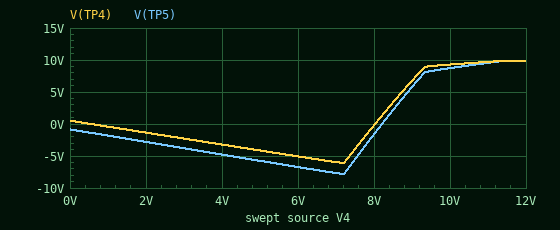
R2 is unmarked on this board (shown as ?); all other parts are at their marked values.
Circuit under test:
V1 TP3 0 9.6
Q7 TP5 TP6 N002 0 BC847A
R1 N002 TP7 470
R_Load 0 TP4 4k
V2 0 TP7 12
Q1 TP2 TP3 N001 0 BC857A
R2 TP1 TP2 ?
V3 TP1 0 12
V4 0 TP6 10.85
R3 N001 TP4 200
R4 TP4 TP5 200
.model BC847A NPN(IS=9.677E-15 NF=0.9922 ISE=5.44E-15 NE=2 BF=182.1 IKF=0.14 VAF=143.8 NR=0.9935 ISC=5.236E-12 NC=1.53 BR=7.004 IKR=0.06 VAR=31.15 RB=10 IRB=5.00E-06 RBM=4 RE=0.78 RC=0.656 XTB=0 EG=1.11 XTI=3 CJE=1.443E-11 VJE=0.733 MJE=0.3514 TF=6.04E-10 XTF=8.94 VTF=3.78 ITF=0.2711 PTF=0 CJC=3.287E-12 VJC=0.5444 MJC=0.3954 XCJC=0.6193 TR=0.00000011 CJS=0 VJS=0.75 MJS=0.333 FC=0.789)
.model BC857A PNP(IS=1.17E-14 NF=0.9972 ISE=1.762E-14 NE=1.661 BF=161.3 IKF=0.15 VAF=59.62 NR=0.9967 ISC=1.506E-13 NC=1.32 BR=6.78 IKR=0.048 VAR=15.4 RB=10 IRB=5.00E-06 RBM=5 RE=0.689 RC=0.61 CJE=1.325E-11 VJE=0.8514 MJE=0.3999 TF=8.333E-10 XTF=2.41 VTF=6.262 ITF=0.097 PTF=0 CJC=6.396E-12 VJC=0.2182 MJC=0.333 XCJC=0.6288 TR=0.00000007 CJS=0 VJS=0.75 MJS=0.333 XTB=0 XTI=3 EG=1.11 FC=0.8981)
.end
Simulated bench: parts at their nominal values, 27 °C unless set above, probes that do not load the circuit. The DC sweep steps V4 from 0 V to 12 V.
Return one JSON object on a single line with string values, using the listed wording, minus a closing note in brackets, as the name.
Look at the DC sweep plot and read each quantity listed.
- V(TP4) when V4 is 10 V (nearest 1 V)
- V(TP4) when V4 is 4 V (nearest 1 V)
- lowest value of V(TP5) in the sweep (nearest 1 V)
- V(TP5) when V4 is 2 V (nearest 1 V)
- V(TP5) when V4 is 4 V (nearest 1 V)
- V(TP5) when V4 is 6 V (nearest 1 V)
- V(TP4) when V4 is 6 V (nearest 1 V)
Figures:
{"V(TP4) when V4 is 10 V": "9 V", "V(TP4) when V4 is 4 V": "-3 V", "lowest value of V(TP5) in the sweep": "-8 V", "V(TP5) when V4 is 2 V": "-3 V", "V(TP5) when V4 is 4 V": "-5 V", "V(TP5) when V4 is 6 V": "-7 V", "V(TP4) when V4 is 6 V": "-5 V"}
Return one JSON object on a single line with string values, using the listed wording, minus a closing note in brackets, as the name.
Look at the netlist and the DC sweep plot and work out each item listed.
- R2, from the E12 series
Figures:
{"R2, from the E12 series": "220 Ω"}
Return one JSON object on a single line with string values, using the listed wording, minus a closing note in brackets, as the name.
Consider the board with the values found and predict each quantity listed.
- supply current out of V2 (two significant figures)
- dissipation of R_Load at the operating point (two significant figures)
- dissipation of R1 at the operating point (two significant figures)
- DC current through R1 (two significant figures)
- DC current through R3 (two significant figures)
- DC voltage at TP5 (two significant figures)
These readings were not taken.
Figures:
{"supply current out of V2": "1.1 mA", "dissipation of R_Load at the operating point": "23 mW", "dissipation of R1 at the operating point": "530 µW", "DC current through R1": "1.1 mA", "DC current through R3": "3.5 mA", "DC voltage at TP5": "9.4 V"}
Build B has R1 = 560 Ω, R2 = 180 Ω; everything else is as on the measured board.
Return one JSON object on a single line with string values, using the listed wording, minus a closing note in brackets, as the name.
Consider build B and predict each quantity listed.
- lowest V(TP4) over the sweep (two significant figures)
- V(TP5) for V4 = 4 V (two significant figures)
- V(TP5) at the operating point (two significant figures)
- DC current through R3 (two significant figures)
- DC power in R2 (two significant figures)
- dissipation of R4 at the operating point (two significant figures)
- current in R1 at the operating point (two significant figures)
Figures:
{"lowest V(TP4) over the sweep": "-4.5 V", "V(TP5) for V4 = 4 V": "-4.7 V", "V(TP5) at the operating point": "9.5 V", "DC current through R3": "3.3 mA", "DC power in R2": "15 mW", "dissipation of R4 at the operating point": "160 µW", "current in R1 at the operating point": "900 µA"}
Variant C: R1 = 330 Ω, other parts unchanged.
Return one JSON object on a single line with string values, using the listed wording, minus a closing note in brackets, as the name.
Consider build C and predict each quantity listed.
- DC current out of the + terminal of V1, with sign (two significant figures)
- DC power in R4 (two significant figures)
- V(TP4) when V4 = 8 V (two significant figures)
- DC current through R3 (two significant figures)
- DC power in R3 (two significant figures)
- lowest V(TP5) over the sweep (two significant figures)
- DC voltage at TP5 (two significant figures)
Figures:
{"DC current out of the + terminal of V1, with sign": "-3.6 mA", "DC power in R4": "440 µW", "V(TP4) when V4 = 8 V": "-6.9 V", "DC current through R3": "3.9 mA", "DC power in R3": "3.0 mW", "lowest V(TP5) over the sweep": "-8.9 V", "DC voltage at TP5": "9.3 V"}
